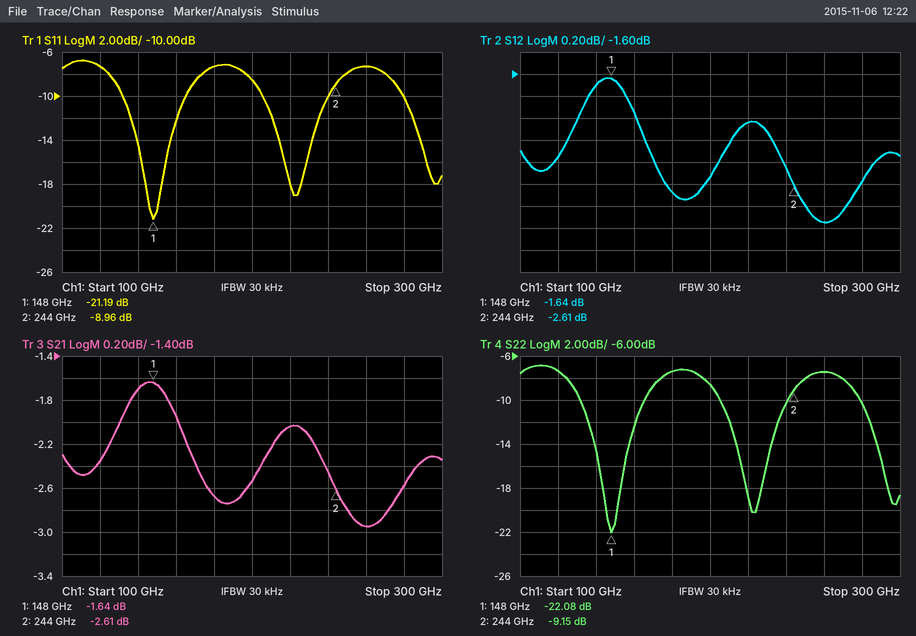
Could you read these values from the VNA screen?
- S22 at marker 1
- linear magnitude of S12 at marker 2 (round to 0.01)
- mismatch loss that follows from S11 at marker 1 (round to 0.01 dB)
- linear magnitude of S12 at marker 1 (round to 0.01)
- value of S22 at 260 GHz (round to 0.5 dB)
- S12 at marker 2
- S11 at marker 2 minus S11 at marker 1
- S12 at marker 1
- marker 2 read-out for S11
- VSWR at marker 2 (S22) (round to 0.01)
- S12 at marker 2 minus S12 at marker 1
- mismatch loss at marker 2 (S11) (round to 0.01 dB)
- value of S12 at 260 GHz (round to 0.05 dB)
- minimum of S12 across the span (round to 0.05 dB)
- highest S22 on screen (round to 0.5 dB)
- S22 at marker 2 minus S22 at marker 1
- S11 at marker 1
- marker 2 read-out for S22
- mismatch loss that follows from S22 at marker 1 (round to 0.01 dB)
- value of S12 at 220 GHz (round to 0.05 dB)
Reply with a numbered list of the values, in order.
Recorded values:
1. -22.08 dB
2. 0.74
3. 0.03 dB
4. 0.83
5. -7.5 dB
6. -2.61 dB
7. 12.23 dB
8. -1.64 dB
9. -8.96 dB
10. 2.07
11. -0.97 dB
12. 0.59 dB
13. -2.95 dB
14. -2.95 dB
15. -7.0 dB
16. 12.93 dB
17. -21.19 dB
18. -9.15 dB
19. 0.03 dB
20. -2.05 dB
